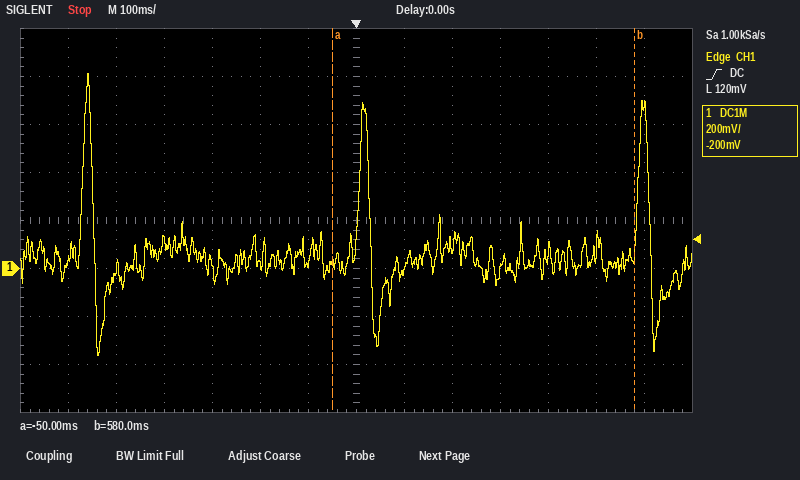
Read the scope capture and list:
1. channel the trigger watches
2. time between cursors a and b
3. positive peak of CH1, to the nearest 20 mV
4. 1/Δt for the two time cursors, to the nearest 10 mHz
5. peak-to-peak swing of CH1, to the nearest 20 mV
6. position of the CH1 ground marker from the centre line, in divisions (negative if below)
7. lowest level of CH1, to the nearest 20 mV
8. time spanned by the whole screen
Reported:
CH1
630 ms
820 mV
1.59 Hz
1.18 V
-1.0 div
-360 mV
1.4 s
